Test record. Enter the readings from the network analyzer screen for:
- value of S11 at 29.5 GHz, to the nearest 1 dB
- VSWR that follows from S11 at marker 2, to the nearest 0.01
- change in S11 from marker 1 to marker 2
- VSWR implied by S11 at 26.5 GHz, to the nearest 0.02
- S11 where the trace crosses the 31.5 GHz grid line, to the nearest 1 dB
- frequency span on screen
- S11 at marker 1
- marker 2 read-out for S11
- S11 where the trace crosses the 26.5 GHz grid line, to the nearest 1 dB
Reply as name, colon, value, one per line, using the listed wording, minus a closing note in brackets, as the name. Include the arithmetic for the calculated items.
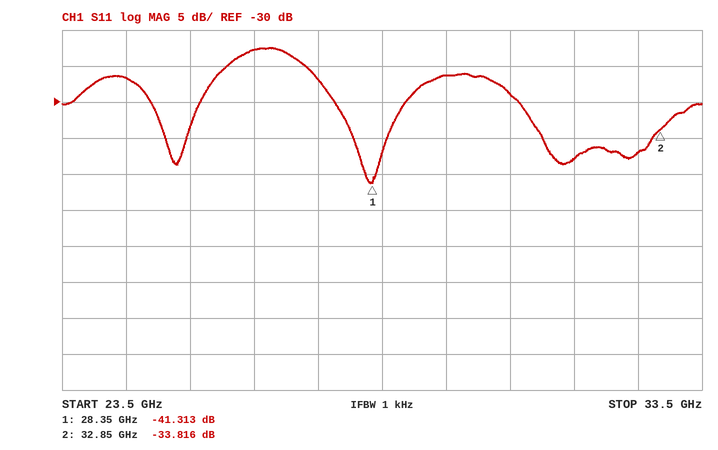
value of S11 at 29.5 GHz, to the nearest 1 dB: -26 dB
VSWR that follows from S11 at marker 2, to the nearest 0.01: (1 + 0.0204)/(1 − 0.0204) ≈ 1.04
change in S11 from marker 1 to marker 2: -33.816 − (-41.313) = 7.497 dB
VSWR implied by S11 at 26.5 GHz, to the nearest 0.02: |Γ| = 10^(-23/20) = 0.0708; VSWR = (1 + 0.0708)/(1 − 0.0708) ≈ 1.15, so 1.16 to the nearest 0.02
S11 where the trace crosses the 31.5 GHz grid line, to the nearest 1 dB: -38 dB
frequency span on screen: 10 GHz
S11 at marker 1: -41.313 dB
marker 2 read-out for S11: -33.816 dB
S11 where the trace crosses the 26.5 GHz grid line, to the nearest 1 dB: -23 dB
